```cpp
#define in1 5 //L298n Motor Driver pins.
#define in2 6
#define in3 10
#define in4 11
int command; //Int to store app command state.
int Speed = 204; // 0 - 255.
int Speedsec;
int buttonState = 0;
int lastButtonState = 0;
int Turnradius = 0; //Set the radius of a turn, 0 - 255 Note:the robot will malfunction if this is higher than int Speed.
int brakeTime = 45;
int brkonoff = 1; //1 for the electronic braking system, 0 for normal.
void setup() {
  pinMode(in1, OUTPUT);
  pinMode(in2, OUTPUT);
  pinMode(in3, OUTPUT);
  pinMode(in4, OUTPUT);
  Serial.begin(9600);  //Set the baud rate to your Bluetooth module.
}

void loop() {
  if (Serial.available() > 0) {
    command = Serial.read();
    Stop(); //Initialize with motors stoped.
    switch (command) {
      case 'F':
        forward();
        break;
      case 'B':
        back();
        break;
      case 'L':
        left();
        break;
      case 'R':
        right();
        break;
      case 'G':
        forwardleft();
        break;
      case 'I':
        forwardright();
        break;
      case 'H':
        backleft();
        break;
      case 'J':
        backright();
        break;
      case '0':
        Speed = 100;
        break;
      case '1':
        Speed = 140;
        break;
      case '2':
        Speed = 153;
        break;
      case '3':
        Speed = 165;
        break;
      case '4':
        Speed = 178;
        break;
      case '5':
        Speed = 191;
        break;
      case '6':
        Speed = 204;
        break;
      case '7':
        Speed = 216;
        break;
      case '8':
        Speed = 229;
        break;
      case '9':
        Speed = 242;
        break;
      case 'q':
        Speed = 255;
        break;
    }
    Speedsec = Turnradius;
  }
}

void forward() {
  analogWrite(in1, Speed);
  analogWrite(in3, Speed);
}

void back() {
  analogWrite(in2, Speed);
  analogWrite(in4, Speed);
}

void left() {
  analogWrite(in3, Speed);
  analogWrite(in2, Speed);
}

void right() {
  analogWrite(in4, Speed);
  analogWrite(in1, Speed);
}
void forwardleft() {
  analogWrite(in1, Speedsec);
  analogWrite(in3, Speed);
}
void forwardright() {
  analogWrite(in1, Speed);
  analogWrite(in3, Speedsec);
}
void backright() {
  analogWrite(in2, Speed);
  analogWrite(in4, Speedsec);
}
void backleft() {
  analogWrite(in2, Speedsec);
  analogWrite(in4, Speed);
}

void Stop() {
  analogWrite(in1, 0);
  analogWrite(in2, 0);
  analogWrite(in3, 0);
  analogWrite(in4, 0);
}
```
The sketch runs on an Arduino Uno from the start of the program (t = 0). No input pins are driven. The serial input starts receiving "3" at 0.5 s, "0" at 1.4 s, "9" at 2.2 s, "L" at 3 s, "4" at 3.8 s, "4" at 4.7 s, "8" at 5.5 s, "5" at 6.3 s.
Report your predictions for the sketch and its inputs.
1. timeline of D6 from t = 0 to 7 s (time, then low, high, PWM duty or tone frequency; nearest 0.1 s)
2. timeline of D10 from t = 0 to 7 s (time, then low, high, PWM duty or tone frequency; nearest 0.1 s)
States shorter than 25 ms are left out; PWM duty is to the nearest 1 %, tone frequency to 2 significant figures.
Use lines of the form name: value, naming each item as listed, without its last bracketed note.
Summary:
timeline of D6 from t = 0 to 7 s: 0 s low; 3 s PWM 95 %; 3.8 s low
timeline of D10 from t = 0 to 7 s: 0 s low; 3 s PWM 95 %; 3.8 s low
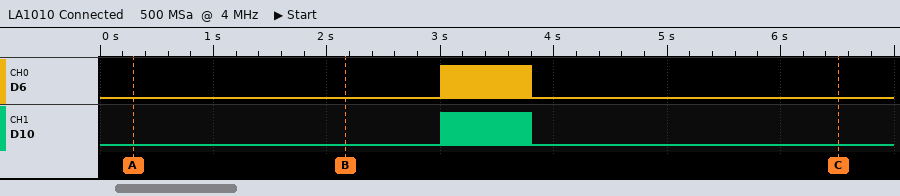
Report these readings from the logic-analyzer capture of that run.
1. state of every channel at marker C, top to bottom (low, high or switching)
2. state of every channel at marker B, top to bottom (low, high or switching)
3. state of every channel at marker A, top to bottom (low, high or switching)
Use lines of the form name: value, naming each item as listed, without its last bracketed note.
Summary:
state of every channel at marker C, top to bottom: D6 low, D10 low
state of every channel at marker B, top to bottom: D6 low, D10 low
state of every channel at marker A, top to bottom: D6 low, D10 low
